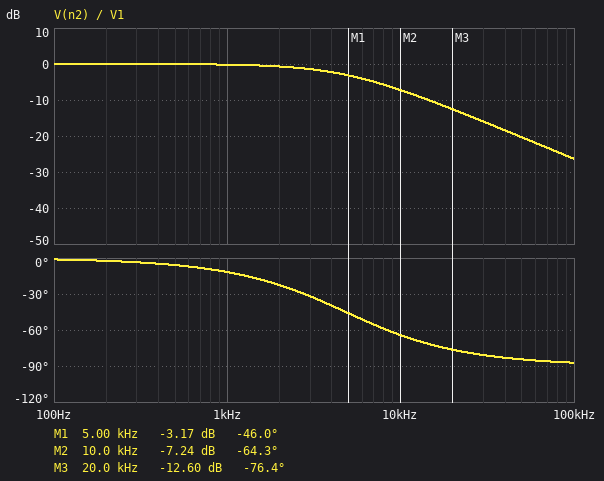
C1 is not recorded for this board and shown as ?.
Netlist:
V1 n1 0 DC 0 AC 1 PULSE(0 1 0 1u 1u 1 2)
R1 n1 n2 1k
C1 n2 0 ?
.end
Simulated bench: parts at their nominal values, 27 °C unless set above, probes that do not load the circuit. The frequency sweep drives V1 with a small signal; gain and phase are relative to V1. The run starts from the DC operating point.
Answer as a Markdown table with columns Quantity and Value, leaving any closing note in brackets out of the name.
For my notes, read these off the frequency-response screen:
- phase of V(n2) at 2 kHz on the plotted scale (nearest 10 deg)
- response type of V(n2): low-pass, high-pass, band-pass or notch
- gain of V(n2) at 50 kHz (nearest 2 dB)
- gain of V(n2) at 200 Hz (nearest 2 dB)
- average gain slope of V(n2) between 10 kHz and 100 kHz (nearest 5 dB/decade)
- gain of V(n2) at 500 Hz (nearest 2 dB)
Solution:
| Quantity | Value |
|---|---|
| phase of V(n2) at 2 kHz on the plotted scale | -20 deg |
| response type of V(n2): low-pass, high-pass, band-pass or notch | low-pass |
| gain of V(n2) at 50 kHz | -20 dB |
| gain of V(n2) at 200 Hz | 0 dB |
| average gain slope of V(n2) between 10 kHz and 100 kHz | -20 dB/decade |
| gain of V(n2) at 500 Hz | 0 dB |
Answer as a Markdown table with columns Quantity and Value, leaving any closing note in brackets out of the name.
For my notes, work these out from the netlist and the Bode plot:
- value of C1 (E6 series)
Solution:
| Quantity | Value |
|---|---|
| value of C1 | 33 nF |
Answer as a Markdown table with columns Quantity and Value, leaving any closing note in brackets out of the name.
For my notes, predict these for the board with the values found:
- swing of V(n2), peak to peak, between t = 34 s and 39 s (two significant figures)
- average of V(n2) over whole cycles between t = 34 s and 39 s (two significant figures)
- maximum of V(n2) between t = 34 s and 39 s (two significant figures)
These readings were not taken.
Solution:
| Quantity | Value |
|---|---|
| swing of V(n2), peak to peak, between t = 34 s and 39 s | 1.0 V |
| average of V(n2) over whole cycles between t = 34 s and 39 s | 500 mV |
| maximum of V(n2) between t = 34 s and 39 s | 1.0 V |
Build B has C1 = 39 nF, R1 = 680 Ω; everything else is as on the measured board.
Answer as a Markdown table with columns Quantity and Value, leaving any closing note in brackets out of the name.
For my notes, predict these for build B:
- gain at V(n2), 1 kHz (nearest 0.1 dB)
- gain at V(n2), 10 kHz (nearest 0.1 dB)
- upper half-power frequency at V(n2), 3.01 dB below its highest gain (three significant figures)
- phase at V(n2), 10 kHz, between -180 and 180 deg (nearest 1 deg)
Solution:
| Quantity | Value |
|---|---|
| gain at V(n2), 1 kHz | -0.1 dB |
| gain at V(n2), 10 kHz | -5.8 dB |
| upper half-power frequency at V(n2), 3.01 dB below its highest gain | 6.00 kHz |
| phase at V(n2), 10 kHz, between -180 and 180 deg | -59 deg |
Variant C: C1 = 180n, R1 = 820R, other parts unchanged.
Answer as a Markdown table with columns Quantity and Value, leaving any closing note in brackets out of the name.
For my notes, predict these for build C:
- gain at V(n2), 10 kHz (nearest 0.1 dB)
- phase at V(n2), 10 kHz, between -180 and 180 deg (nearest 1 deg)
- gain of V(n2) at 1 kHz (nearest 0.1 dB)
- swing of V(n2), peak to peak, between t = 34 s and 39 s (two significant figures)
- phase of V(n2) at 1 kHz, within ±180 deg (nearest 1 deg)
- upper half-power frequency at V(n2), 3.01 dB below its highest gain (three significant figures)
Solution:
| Quantity | Value |
|---|---|
| gain at V(n2), 10 kHz | -19.4 dB |
| phase at V(n2), 10 kHz, between -180 and 180 deg | -84 deg |
| gain of V(n2) at 1 kHz | -2.7 dB |
| swing of V(n2), peak to peak, between t = 34 s and 39 s | 1.0 V |
| phase of V(n2) at 1 kHz, within ±180 deg | -43 deg |
| upper half-power frequency at V(n2), 3.01 dB below its highest gain | 1.08 kHz |
